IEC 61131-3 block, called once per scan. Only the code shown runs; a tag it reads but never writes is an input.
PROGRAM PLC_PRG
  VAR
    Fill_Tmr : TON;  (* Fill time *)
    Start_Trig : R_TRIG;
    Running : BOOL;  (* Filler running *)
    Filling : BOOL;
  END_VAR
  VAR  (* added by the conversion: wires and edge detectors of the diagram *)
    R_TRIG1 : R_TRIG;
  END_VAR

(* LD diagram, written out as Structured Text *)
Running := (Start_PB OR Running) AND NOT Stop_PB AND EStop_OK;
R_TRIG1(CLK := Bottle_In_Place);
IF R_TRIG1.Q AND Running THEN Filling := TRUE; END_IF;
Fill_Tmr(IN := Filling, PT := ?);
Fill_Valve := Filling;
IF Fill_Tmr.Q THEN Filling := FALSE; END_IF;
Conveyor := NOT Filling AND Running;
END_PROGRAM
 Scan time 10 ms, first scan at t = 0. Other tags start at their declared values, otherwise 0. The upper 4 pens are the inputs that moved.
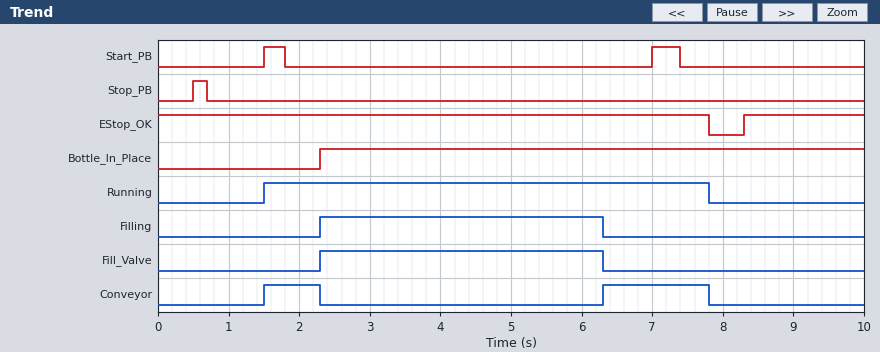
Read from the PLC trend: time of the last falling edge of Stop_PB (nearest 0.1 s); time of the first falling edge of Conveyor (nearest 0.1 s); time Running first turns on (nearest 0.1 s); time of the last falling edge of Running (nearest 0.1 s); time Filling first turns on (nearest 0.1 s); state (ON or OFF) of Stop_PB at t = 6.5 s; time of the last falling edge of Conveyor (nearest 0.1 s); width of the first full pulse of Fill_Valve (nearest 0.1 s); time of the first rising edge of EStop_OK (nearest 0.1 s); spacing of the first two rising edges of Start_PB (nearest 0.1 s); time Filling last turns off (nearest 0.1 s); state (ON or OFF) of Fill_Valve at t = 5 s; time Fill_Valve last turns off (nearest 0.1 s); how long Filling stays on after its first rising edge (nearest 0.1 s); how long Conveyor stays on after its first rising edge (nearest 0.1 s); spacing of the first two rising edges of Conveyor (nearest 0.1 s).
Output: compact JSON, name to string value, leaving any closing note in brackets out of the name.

{"time of the last falling edge of Stop_PB": "0.7 s", "time of the first falling edge of Conveyor": "2.3 s", "time Running first turns on": "1.5 s", "time of the last falling edge of Running": "7.8 s", "time Filling first turns on": "2.3 s", "state (ON or OFF) of Stop_PB at t = 6.5 s": "OFF", "time of the last falling edge of Conveyor": "7.8 s", "width of the first full pulse of Fill_Valve": "4.0 s", "time of the first rising edge of EStop_OK": "8.3 s", "spacing of the first two rising edges of Start_PB": "5.5 s", "time Filling last turns off": "6.3 s", "state (ON or OFF) of Fill_Valve at t = 5 s": "ON", "time Fill_Valve last turns off": "6.3 s", "how long Filling stays on after its first rising edge": "4.0 s", "how long Conveyor stays on after its first rising edge": "0.8 s", "spacing of the first two rising edges of Conveyor": "4.8 s"}
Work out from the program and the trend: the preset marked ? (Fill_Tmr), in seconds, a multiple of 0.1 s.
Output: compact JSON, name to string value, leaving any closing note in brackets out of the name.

{"the preset marked ? (Fill_Tmr), in seconds, a multiple of 0.1 s": "4.0 s"}
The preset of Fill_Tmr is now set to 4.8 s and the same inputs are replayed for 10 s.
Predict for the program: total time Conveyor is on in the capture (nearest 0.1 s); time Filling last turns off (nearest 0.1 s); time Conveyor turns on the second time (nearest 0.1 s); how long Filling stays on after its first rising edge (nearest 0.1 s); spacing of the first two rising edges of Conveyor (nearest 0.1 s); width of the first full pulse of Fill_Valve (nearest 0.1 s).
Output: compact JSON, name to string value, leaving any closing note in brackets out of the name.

{"total time Conveyor is on in the capture": "1.5 s", "time Filling last turns off": "7.1 s", "time Conveyor turns on the second time": "7.1 s", "how long Filling stays on after its first rising edge": "4.8 s", "spacing of the first two rising edges of Conveyor": "5.6 s", "width of the first full pulse of Fill_Valve": "4.8 s"}
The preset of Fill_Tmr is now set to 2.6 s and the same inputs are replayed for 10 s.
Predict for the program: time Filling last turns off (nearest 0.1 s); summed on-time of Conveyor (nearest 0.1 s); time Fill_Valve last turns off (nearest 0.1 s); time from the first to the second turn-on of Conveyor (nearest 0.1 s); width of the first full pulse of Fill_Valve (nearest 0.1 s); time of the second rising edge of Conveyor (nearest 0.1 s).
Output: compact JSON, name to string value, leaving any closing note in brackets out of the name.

{"time Filling last turns off": "4.9 s", "summed on-time of Conveyor": "3.7 s", "time Fill_Valve last turns off": "4.9 s", "time from the first to the second turn-on of Conveyor": "3.4 s", "width of the first full pulse of Fill_Valve": "2.6 s", "time of the second rising edge of Conveyor": "4.9 s"}
